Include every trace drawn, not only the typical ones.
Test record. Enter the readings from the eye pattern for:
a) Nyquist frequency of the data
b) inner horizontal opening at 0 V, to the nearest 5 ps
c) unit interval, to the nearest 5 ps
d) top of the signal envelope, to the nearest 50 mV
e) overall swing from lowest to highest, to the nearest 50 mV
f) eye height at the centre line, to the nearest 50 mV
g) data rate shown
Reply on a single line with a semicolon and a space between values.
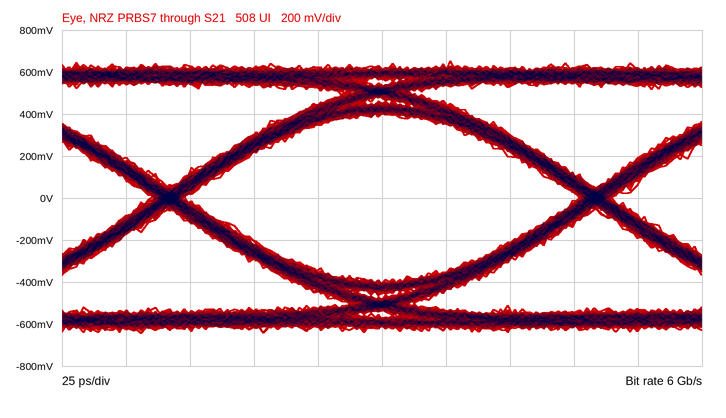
3 GHz; 155 ps; 165 ps; 650 mV; 1.30 V; 800 mV; 6 Gb/s
